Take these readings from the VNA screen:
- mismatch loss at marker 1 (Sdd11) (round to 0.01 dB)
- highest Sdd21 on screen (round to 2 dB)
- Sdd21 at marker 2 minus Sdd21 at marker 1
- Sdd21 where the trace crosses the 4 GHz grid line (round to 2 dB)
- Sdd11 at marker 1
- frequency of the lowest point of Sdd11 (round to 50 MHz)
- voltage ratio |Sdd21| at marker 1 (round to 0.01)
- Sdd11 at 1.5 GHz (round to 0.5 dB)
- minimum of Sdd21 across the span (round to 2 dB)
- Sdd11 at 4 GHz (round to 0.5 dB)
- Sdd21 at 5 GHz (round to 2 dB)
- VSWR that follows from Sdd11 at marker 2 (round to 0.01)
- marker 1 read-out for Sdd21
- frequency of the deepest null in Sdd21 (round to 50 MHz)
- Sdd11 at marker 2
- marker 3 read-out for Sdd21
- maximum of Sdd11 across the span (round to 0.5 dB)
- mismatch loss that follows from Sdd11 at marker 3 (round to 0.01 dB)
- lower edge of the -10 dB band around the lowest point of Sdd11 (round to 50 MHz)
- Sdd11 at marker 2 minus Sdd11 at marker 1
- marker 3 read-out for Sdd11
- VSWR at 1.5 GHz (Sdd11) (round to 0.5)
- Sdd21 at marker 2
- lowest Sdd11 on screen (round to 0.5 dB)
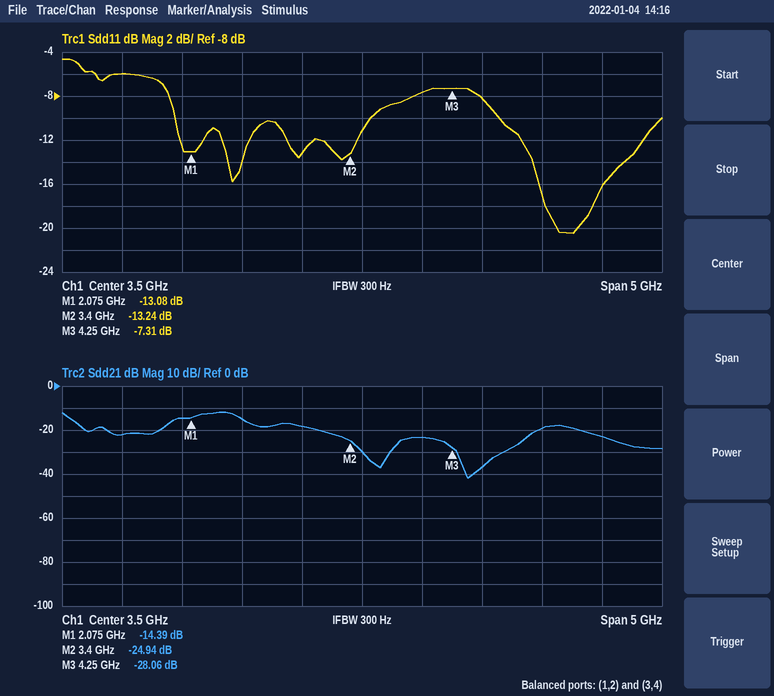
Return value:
0.22 dB
-12 dB
-10.55 dB
-24 dB
-13.08 dB
5.25 GHz
0.19
-6.0 dB
-42 dB
-7.5 dB
-20 dB
1.56
-14.39 dB
4.40 GHz
-13.24 dB
-28.06 dB
-4.5 dB
0.89 dB
4.65 GHz
-0.16 dB
-7.31 dB
3.0
-24.94 dB
-20.5 dB
